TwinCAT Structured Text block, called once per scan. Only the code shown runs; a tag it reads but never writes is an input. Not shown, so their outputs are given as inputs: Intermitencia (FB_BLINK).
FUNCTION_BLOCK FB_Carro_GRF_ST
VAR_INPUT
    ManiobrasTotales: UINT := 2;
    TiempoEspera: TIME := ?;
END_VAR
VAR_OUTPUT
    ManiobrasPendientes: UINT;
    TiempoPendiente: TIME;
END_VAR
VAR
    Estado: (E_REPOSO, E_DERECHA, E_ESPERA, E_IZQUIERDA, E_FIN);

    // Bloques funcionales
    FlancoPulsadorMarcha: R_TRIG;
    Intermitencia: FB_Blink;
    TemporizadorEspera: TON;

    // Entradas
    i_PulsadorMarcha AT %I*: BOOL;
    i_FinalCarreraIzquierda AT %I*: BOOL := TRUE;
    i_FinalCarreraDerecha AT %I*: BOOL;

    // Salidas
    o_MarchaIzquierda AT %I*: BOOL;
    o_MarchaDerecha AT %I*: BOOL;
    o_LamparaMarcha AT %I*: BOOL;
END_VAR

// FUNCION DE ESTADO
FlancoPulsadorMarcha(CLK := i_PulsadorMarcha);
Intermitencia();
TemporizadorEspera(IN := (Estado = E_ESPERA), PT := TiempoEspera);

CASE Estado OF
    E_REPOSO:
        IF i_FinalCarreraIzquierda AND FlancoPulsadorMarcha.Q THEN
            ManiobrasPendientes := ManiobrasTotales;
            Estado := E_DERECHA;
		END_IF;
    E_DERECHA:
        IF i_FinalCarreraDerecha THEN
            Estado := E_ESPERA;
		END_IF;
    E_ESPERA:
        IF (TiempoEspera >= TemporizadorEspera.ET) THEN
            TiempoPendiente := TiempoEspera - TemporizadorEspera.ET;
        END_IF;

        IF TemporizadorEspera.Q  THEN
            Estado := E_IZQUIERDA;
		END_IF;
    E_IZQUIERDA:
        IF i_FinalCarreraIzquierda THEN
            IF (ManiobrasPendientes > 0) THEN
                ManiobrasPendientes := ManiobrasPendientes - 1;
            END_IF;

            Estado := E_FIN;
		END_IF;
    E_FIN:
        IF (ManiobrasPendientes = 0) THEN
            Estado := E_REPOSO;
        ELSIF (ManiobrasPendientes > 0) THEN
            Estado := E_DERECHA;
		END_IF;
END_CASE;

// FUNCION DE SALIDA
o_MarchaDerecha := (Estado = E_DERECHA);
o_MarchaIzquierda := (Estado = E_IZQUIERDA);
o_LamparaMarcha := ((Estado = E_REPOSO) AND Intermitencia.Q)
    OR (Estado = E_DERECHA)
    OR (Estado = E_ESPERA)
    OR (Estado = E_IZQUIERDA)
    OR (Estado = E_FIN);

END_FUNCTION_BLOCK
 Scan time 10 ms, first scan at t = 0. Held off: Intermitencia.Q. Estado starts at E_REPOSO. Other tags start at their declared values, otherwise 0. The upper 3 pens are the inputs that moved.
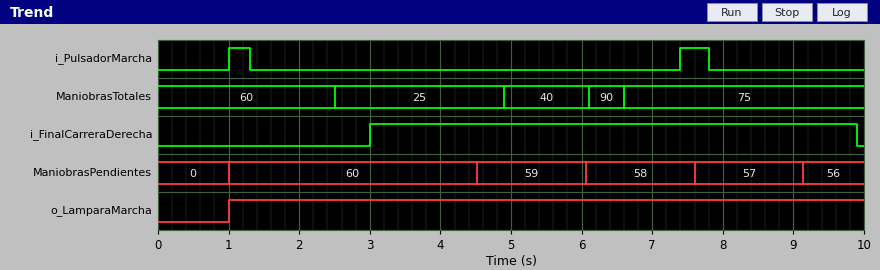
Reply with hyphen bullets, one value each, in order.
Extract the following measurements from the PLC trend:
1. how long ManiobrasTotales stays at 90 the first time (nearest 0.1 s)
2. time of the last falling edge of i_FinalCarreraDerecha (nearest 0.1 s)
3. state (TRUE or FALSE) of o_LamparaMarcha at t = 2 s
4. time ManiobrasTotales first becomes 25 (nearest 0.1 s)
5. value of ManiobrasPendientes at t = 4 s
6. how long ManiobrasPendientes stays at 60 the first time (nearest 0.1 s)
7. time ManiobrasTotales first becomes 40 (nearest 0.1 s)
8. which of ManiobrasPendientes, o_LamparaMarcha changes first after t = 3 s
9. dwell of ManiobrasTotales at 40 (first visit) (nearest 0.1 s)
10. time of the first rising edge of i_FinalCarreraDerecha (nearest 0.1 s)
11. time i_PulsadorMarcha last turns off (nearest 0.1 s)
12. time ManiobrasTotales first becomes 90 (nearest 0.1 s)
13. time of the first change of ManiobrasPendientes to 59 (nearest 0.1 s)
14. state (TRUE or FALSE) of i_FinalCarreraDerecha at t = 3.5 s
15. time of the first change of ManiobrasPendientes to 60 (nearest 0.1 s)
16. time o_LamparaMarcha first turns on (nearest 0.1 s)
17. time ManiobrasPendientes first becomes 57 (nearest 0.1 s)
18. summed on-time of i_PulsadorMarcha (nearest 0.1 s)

- 0.5 s
- 9.9 s
- TRUE
- 2.5 s
- 60
- 3.5 s
- 4.9 s
- ManiobrasPendientes
- 1.2 s
- 3.0 s
- 7.8 s
- 6.1 s
- 4.5 s
- TRUE
- 1.0 s
- 1.0 s
- 7.6 s
- 0.7 s
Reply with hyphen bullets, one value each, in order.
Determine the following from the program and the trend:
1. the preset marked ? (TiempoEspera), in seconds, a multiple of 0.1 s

- 1.5 s
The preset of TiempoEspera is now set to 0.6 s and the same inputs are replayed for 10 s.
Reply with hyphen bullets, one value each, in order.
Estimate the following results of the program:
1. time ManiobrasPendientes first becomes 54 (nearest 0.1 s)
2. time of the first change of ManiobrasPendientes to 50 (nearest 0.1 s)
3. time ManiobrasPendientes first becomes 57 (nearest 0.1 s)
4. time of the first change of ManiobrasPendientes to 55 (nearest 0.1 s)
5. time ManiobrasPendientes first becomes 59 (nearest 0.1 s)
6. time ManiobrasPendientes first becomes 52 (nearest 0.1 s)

- 6.8 s
- 9.4 s
- 4.9 s
- 6.2 s
- 3.6 s
- 8.1 s
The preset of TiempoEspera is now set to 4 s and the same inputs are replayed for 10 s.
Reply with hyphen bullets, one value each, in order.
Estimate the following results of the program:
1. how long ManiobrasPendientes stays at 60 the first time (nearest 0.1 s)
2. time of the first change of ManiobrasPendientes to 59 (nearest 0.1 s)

- 6.0 s
- 7.0 s
